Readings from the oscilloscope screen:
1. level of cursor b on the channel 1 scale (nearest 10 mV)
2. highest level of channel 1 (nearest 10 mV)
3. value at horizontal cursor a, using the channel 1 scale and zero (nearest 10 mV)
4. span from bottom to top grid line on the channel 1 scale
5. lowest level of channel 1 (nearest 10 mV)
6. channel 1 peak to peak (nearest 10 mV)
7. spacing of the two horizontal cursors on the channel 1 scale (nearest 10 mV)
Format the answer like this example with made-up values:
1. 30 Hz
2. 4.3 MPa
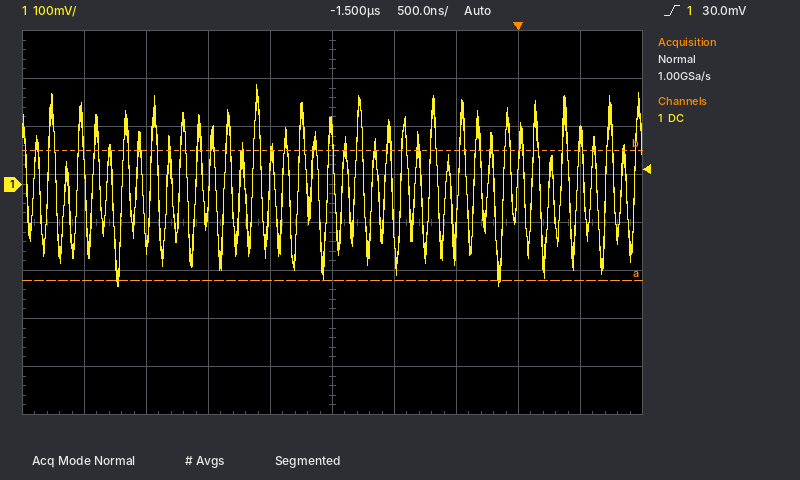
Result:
1. 70 mV
2. 210 mV
3. -200 mV
4. 800 mV
5. -210 mV
6. 420 mV
7. 270 mV
